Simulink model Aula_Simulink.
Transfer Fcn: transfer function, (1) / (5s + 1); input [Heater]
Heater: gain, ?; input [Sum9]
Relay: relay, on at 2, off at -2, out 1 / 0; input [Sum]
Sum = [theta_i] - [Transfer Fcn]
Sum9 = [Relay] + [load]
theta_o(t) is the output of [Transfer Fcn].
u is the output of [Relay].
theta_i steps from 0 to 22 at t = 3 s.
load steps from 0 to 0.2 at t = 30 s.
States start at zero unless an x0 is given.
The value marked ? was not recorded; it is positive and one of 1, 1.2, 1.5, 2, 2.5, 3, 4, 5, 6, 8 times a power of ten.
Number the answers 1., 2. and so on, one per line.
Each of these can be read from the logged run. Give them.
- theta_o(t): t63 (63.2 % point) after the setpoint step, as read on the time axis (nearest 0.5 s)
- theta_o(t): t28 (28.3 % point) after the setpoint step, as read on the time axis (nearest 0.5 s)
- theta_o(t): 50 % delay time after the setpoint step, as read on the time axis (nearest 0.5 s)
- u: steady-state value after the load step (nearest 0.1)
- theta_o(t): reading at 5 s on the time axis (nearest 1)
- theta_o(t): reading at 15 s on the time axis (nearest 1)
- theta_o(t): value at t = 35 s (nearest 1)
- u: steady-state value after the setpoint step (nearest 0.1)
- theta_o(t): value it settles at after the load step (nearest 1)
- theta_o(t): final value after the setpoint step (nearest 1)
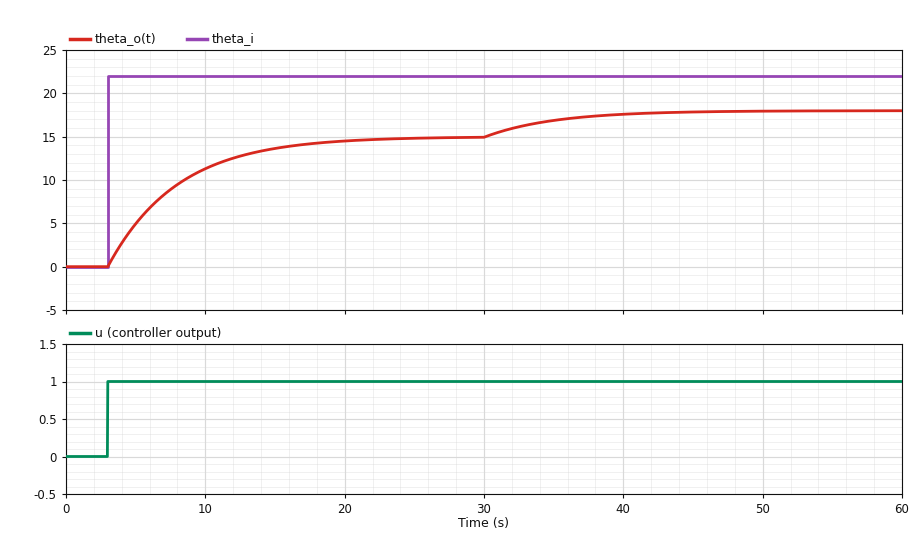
1. 8.0 s
2. 4.5 s
3. 6.5 s
4. 1.0
5. 5
6. 14
7. 17
8. 1.0
9. 18
10. 15
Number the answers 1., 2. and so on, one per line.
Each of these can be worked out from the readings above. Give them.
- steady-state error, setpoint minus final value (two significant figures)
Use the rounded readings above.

1. 7.0
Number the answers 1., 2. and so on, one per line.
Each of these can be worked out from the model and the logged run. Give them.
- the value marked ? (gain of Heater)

1. 15
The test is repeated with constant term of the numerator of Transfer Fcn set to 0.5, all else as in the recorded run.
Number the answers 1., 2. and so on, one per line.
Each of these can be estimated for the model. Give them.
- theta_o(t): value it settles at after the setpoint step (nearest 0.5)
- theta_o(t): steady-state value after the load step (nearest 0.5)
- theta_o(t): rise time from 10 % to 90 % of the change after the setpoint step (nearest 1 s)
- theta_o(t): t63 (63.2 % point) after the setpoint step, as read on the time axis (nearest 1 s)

1. 7.5
2. 9.0
3. 11 s
4. 8 s
